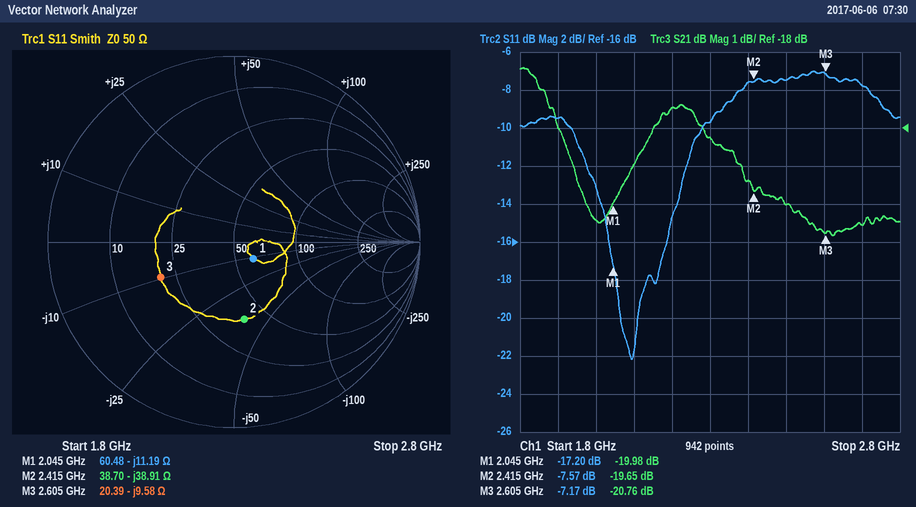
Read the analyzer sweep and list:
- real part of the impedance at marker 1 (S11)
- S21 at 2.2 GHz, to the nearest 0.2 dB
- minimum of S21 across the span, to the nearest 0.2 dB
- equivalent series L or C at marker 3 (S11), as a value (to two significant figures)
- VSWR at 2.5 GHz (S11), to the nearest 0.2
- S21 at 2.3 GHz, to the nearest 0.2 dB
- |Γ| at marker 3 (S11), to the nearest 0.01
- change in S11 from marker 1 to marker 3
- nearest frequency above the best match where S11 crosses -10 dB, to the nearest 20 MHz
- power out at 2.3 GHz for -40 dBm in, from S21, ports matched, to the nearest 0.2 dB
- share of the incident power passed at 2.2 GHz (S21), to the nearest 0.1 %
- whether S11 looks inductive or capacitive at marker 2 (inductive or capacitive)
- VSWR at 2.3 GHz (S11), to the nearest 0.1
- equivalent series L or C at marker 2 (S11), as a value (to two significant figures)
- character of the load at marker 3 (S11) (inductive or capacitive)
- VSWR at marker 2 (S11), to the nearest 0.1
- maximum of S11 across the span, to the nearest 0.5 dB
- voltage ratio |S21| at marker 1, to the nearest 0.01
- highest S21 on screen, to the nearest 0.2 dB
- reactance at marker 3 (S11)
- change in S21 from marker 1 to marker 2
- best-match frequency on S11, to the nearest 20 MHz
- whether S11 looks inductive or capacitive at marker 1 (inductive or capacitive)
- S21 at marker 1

60.48 Ω
-17.4 dB
-20.8 dB
6.4 pF
2.4
-18.2 dB
0.44
10.03 dB
2.28 GHz
-58.2 dBm
1.8 %
capacitive
2.0
1.7 pF
capacitive
2.4
-7.0 dB
0.10
-16.4 dB
-9.58 Ω
0.33 dB
2.10 GHz
capacitive
-19.98 dB
